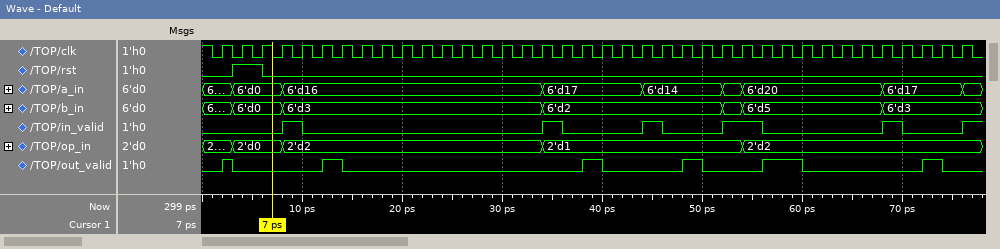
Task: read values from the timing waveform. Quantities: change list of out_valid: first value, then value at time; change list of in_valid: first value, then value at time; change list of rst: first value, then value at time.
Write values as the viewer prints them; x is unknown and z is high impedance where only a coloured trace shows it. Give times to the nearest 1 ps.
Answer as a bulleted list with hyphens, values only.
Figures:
- 0, 1 at 2 ps, 0 at 3 ps, 1 at 12 ps, 0 at 14 ps, 1 at 38 ps, 0 at 40 ps, 1 at 48 ps, 0 at 50 ps, 1 at 56 ps, 0 at 60 ps, 1 at 72 ps, 0 at 74 ps
- 0, 1 at 8 ps, 0 at 10 ps, 1 at 34 ps, 0 at 36 ps, 1 at 44 ps, 0 at 46 ps, 1 at 52 ps, 0 at 56 ps, 1 at 68 ps, 0 at 70 ps, 1 at 76 ps
- 0, 1 at 3 ps, 0 at 6 ps
